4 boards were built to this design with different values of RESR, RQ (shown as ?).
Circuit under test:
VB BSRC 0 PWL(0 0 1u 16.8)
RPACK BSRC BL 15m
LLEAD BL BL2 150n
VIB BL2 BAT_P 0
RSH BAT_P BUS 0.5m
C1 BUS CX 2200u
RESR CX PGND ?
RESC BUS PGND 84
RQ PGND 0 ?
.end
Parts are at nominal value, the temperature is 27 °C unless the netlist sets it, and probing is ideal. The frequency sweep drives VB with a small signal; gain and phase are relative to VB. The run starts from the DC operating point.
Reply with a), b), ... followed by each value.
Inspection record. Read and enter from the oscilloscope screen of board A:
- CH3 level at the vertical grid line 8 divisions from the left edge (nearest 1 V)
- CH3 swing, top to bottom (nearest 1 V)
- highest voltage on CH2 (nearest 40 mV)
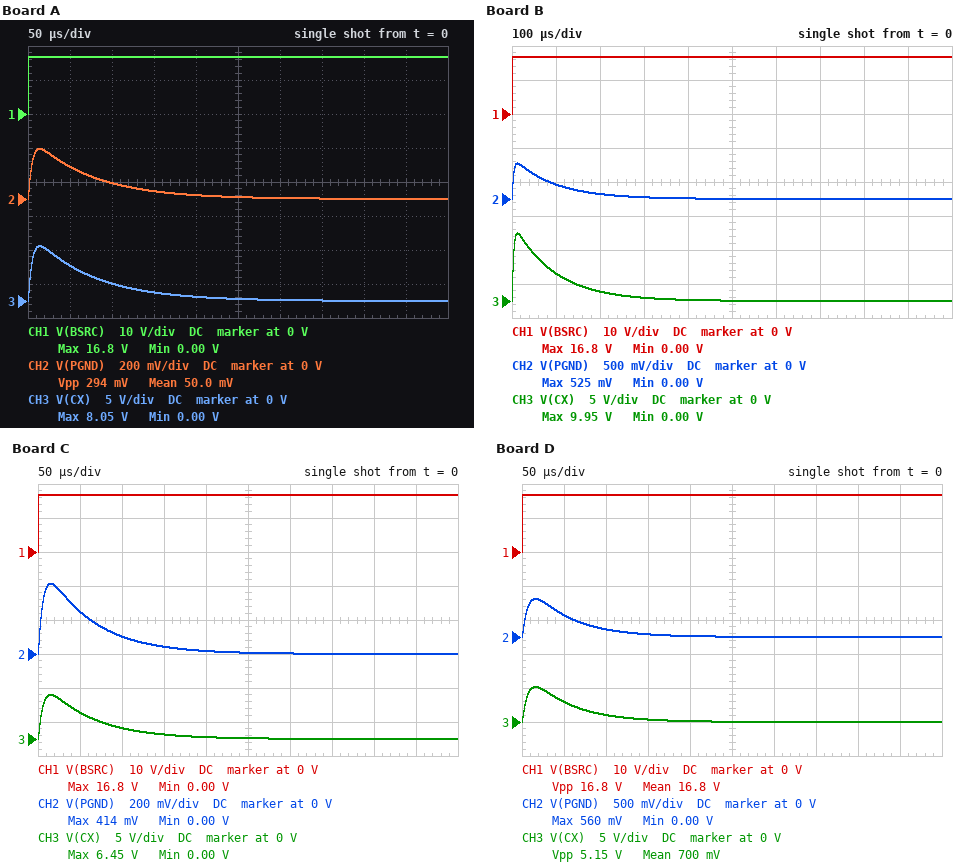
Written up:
a) 0 V
b) 8 V
c) 280 mV
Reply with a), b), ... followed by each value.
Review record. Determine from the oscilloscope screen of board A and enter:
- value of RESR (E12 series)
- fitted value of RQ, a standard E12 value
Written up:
a) 0.018 Ω
b) 680 µΩ
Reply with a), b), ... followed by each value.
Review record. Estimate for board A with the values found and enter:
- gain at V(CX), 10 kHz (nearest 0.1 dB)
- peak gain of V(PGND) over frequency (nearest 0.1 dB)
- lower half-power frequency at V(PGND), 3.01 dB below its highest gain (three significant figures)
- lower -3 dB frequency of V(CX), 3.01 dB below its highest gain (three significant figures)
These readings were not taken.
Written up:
a) -5.3 dB
b) -34.0 dB
c) 2.01 kHz
d) 2.01 kHz
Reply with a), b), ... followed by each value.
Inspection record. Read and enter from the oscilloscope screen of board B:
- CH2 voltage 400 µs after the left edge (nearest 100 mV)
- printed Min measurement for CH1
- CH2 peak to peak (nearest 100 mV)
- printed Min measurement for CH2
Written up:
a) 0 V
b) 0.00 V
c) 500 mV
d) 0.00 V
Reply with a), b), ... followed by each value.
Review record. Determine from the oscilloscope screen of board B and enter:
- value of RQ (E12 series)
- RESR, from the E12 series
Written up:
a) 1.5 mΩ
b) 0.027 Ω
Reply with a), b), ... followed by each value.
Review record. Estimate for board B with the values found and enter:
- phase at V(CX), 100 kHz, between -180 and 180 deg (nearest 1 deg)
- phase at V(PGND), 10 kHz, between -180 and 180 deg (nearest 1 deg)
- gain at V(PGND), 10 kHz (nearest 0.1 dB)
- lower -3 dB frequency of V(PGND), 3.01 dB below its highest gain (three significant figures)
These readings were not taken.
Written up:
a) -65 deg
b) -3 deg
c) -29.4 dB
d) 1.59 kHz
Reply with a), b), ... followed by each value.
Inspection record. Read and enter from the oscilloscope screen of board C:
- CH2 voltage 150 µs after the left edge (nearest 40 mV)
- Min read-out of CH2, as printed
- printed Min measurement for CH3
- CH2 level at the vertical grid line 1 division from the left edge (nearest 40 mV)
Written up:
a) 40 mV
b) 0.00 V
c) 0.00 V
d) 240 mV
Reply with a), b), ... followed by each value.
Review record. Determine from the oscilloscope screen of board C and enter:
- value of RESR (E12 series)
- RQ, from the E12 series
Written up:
a) 0.012 Ω
b) 820 µΩ
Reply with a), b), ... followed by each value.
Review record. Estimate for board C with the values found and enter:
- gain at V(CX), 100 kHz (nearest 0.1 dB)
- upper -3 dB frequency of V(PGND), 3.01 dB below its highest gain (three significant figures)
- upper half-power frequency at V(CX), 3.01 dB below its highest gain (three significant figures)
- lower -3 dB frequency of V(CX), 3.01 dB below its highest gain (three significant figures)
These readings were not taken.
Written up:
a) -17.6 dB
b) 32.4 kHz
c) 32.4 kHz
d) 2.37 kHz
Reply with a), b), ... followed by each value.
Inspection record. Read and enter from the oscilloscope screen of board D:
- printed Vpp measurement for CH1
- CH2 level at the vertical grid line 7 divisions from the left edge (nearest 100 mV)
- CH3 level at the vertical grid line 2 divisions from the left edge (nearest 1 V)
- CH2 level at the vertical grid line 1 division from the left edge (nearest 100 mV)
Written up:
a) 16.8 V
b) 0 V
c) 1 V
d) 300 mV
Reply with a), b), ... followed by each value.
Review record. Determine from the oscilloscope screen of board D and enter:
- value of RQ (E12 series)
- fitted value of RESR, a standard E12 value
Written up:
a) 1 mΩ
b) 8.2 mΩ
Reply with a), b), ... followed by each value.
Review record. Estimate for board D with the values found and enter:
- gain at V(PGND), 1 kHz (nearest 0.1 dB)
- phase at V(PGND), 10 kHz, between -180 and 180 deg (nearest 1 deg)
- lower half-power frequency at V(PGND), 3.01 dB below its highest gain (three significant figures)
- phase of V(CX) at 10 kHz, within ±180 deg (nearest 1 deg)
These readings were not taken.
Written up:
a) -37.6 dB
b) -5 deg
c) 2.66 kHz
d) -5 deg
